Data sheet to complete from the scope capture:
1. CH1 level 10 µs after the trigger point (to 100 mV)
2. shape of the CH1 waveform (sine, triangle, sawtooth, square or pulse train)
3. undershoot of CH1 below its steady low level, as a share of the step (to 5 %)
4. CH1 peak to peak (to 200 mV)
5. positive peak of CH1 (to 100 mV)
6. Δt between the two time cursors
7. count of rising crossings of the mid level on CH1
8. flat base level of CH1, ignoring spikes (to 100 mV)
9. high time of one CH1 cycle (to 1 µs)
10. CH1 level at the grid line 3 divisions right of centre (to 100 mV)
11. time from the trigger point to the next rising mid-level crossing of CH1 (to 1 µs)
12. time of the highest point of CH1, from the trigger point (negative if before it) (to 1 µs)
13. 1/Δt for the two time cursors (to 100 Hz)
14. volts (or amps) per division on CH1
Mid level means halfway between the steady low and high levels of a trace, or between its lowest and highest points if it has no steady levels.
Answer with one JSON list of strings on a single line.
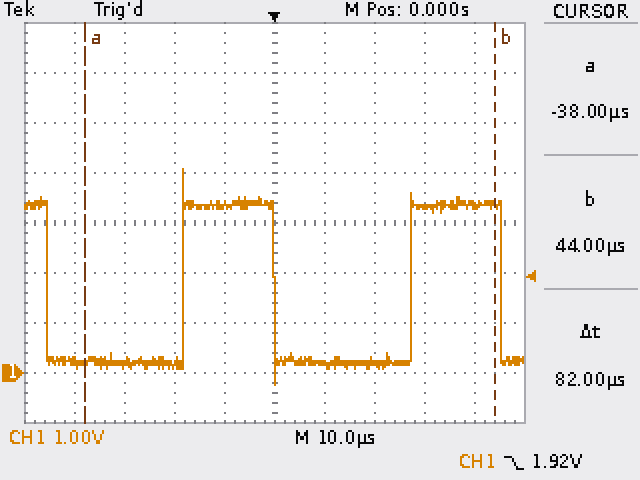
["200 mV", "pulse train", "15 %", "4.4 V", "4.1 V", "82 µs", "2", "200 mV", "18 µs", "3.3 V", "27 µs", "-18 µs", "12.2 kHz", "1 V"]
